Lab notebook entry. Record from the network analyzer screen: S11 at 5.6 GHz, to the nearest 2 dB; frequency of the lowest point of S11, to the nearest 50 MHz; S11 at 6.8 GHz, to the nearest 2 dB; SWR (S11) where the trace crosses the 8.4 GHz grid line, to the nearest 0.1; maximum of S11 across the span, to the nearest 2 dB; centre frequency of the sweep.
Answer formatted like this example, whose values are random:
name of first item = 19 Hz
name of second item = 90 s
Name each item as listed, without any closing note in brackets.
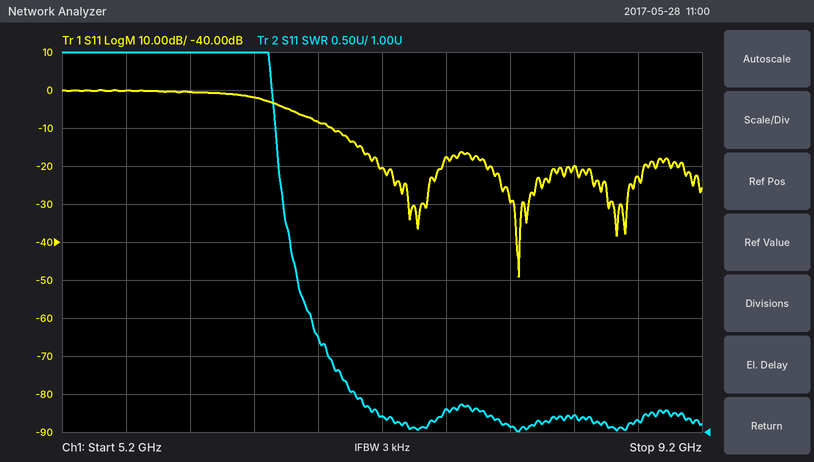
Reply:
S11 at 5.6 GHz, to the nearest 2 dB = 0 dB
frequency of the lowest point of S11, to the nearest 50 MHz = 8.05 GHz
S11 at 6.8 GHz, to the nearest 2 dB = -8 dB
SWR (S11) where the trace crosses the 8.4 GHz grid line, to the nearest 0.1 = 1.2
maximum of S11 across the span, to the nearest 2 dB = 0 dB
centre frequency of the sweep = 7.2 GHz
